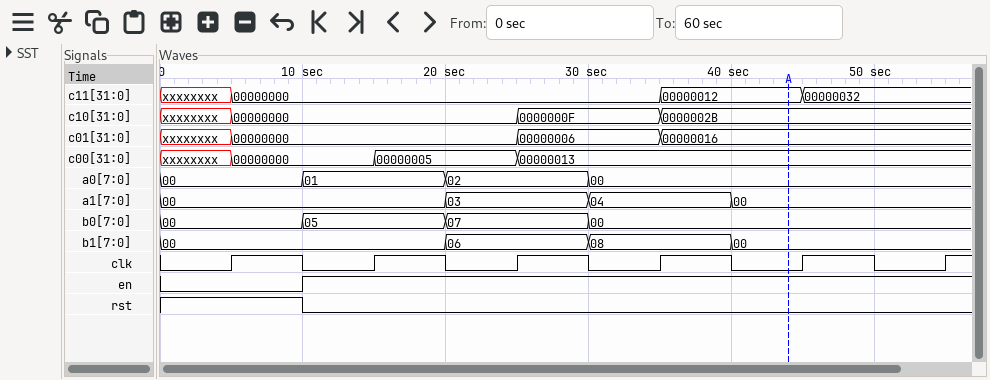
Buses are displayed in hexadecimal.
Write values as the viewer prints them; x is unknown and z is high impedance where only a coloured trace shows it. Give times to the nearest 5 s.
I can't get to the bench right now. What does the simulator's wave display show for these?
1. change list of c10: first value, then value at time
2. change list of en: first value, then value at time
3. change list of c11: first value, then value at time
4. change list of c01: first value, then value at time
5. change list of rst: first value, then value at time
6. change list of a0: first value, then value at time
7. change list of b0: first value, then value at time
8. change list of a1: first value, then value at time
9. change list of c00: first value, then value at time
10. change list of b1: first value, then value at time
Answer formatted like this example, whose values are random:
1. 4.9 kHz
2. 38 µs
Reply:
1. xxxxxxxx, 00000000 at 5 s, 0000000F at 25 s, 0000002B at 35 s
2. 0, 1 at 10 s
3. xxxxxxxx, 00000000 at 5 s, 00000012 at 35 s, 00000032 at 45 s
4. xxxxxxxx, 00000000 at 5 s, 00000006 at 25 s, 00000016 at 35 s
5. 1, 0 at 10 s
6. 00, 01 at 10 s, 02 at 20 s, 00 at 30 s
7. 00, 05 at 10 s, 07 at 20 s, 00 at 30 s
8. 00, 03 at 20 s, 04 at 30 s, 00 at 40 s
9. xxxxxxxx, 00000000 at 5 s, 00000005 at 15 s, 00000013 at 25 s
10. 00, 06 at 20 s, 08 at 30 s, 00 at 40 s
